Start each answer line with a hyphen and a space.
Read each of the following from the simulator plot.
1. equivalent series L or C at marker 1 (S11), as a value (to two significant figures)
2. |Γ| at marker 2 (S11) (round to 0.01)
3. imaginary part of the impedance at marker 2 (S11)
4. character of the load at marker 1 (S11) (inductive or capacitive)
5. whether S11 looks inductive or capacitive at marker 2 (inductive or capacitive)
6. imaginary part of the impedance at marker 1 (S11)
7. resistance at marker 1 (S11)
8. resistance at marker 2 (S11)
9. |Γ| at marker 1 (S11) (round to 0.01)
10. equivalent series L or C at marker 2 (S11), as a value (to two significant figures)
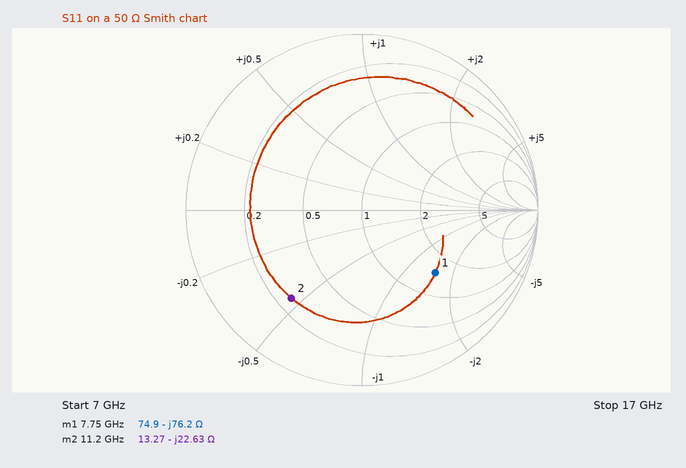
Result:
- 270 fF
- 0.64
- -22.63 Ω
- capacitive
- capacitive
- -76.2 Ω
- 74.9 Ω
- 13.27 Ω
- 0.55
- 630 fF
